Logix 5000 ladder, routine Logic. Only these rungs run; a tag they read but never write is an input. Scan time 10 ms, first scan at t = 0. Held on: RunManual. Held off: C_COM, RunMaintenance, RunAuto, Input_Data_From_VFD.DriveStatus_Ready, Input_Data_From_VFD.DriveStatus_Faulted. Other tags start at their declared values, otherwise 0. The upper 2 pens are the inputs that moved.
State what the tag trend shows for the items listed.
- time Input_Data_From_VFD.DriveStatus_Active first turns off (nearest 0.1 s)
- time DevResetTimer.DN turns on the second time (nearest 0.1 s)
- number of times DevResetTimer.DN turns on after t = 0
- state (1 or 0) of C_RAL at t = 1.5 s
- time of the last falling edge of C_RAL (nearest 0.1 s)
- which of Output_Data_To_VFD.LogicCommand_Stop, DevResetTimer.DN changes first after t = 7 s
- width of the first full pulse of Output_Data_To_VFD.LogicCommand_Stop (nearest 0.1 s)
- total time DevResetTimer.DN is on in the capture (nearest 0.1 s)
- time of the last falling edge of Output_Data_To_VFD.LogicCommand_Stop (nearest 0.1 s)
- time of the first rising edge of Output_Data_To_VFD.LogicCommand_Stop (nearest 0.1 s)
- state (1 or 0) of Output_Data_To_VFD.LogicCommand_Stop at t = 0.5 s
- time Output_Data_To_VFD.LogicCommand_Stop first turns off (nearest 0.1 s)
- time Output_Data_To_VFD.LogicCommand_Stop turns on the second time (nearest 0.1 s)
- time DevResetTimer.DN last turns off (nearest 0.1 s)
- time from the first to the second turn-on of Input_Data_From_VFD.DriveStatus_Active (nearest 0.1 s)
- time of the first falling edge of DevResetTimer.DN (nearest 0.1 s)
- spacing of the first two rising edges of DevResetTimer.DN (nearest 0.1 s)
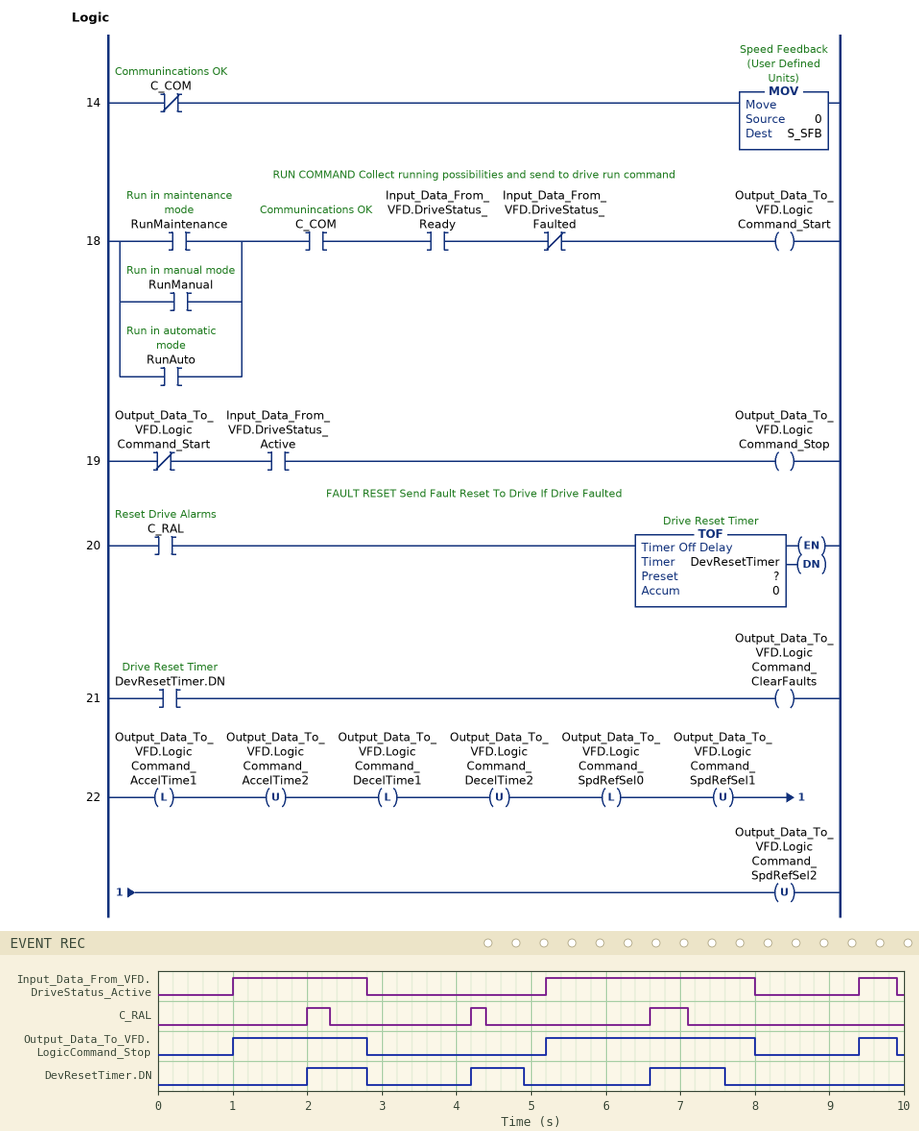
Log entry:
2.8 s
4.2 s
3
0
7.1 s
DevResetTimer.DN
1.8 s
2.5 s
9.9 s
1.0 s
0
2.8 s
5.2 s
7.6 s
4.2 s
2.8 s
2.2 s
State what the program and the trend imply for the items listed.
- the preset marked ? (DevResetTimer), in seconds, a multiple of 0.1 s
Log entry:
0.5 s
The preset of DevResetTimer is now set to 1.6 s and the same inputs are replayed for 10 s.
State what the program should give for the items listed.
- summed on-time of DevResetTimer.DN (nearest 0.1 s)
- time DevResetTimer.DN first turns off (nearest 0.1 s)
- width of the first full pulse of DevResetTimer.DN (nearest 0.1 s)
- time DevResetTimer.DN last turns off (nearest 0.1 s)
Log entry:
5.8 s
3.9 s
1.9 s
8.7 s
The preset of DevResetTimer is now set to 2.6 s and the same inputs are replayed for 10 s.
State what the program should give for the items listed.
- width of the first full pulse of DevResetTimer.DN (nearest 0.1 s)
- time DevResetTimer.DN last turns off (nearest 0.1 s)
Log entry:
7.7 s
9.7 s
